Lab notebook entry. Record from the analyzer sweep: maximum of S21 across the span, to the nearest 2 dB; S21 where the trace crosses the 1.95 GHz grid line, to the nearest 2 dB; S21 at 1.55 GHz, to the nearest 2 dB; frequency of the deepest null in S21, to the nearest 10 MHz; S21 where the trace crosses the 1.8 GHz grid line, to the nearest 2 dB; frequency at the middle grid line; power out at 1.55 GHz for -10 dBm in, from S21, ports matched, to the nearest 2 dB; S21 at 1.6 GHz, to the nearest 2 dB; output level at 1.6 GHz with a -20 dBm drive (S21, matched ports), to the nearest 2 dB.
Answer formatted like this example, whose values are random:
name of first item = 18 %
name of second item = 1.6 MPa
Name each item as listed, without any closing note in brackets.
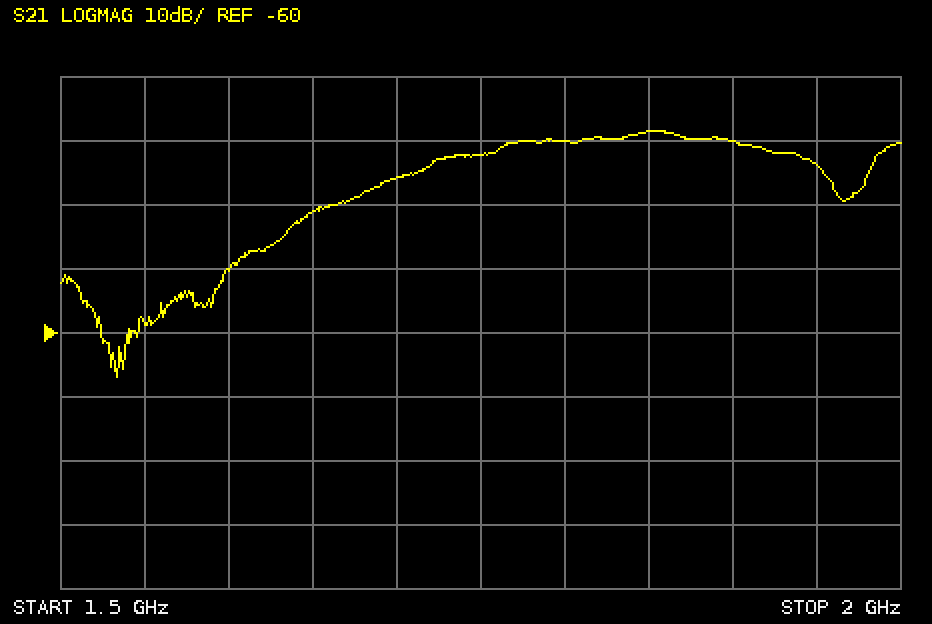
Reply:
maximum of S21 across the span, to the nearest 2 dB = -28 dB
S21 where the trace crosses the 1.95 GHz grid line, to the nearest 2 dB = -34 dB
S21 at 1.55 GHz, to the nearest 2 dB = -58 dB
frequency of the deepest null in S21, to the nearest 10 MHz = 1.53 GHz
S21 where the trace crosses the 1.8 GHz grid line, to the nearest 2 dB = -30 dB
frequency at the middle grid line = 1.75 GHz
power out at 1.55 GHz for -10 dBm in, from S21, ports matched, to the nearest 2 dB = -68 dBm
S21 at 1.6 GHz, to the nearest 2 dB = -50 dB
output level at 1.6 GHz with a -20 dBm drive (S21, matched ports), to the nearest 2 dB = -70 dBm
